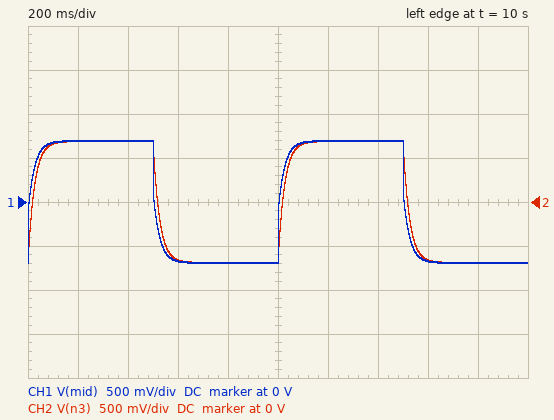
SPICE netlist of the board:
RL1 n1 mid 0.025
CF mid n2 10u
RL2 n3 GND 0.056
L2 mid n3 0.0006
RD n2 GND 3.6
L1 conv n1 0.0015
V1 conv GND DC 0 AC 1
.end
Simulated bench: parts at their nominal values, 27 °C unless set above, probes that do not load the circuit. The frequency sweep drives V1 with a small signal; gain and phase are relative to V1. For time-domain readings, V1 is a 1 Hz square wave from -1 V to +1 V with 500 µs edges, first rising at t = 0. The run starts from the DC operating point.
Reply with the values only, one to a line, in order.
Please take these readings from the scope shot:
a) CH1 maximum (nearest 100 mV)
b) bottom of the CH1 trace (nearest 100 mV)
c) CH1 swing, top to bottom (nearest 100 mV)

700 mV
-700 mV
1.4 V
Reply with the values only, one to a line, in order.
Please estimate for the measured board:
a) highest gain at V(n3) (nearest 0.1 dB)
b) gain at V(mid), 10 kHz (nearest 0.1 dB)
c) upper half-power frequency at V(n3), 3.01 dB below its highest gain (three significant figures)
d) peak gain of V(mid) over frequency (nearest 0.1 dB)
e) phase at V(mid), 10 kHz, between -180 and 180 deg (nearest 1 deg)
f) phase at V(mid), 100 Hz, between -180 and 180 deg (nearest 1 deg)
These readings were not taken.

-3.2 dB
-27.1 dB
6.14 Hz
-3.2 dB
-106 deg
-5 deg
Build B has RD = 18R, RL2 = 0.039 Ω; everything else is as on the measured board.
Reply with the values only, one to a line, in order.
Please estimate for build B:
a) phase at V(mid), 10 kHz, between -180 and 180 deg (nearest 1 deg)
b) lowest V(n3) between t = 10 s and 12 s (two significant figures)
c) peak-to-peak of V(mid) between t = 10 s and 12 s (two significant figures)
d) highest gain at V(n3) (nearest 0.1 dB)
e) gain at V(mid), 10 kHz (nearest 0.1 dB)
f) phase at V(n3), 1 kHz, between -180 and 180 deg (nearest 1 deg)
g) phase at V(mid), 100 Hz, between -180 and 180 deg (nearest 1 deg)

-60 deg
-610 mV
1.2 V
-4.3 dB
-15.6 dB
-95 deg
-3 deg
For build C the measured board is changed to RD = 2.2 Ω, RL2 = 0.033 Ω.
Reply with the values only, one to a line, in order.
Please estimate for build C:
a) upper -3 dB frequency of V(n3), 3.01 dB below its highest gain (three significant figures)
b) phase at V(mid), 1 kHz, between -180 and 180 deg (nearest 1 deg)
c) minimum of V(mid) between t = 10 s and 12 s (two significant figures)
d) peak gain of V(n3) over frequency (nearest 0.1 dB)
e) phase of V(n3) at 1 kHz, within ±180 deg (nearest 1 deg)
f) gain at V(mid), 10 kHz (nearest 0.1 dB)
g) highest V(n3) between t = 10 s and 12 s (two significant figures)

4.40 Hz
-2 deg
-570 mV
-4.9 dB
-91 deg
-30.3 dB
570 mV
